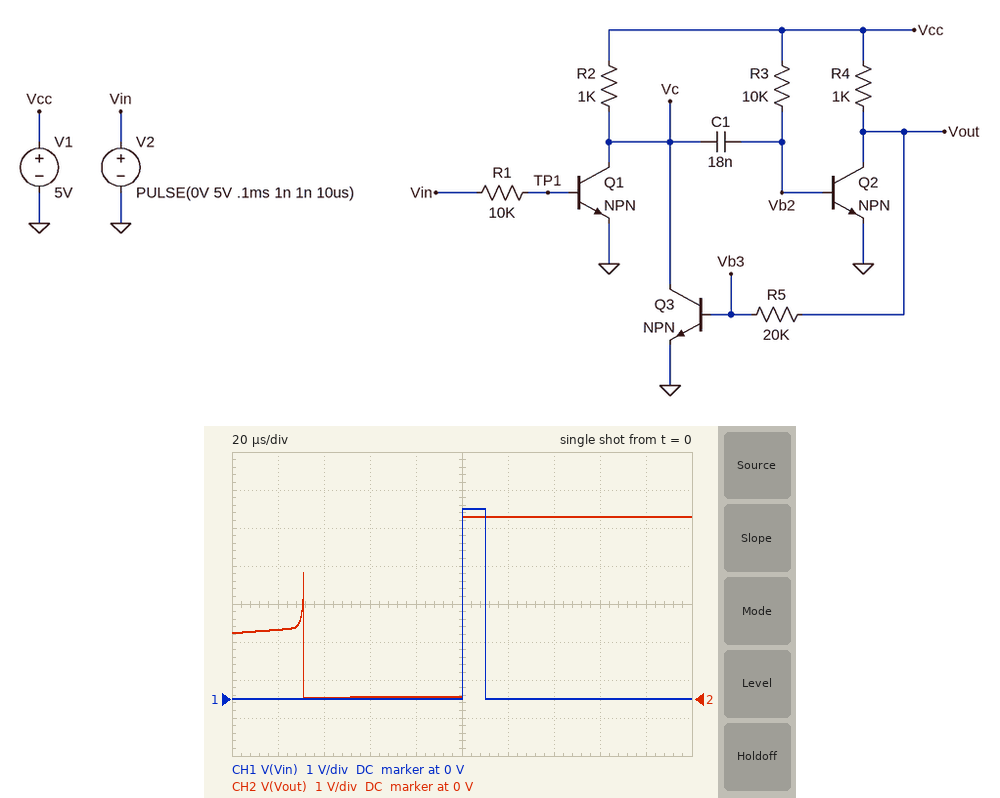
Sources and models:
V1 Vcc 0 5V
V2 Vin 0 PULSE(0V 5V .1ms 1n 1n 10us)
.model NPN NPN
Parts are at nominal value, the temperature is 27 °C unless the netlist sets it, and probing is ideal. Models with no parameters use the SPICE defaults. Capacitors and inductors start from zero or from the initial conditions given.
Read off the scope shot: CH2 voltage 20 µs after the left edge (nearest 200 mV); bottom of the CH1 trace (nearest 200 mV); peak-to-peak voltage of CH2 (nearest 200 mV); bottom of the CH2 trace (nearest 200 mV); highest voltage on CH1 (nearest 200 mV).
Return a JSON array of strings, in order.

["1.8 V", "0 V", "4.8 V", "0 V", "5.0 V"]
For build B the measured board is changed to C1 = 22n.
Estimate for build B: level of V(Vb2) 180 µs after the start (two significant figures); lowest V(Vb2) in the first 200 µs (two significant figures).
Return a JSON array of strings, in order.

["-1.1 V", "-3.8 V"]
